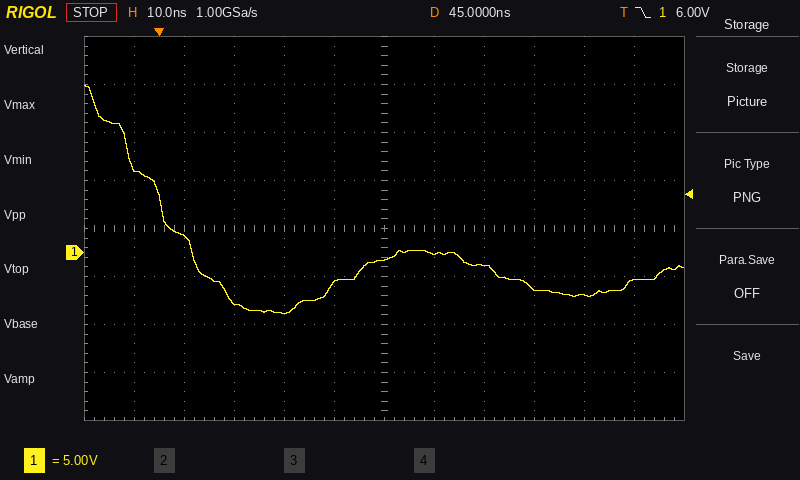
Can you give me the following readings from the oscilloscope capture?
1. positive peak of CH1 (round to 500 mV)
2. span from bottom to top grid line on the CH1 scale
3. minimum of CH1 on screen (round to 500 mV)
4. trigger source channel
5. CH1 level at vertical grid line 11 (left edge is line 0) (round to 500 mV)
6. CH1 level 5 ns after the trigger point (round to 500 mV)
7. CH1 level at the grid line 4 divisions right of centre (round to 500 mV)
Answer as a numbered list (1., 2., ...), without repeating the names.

1. 17.5 V
2. 40 V
3. -6.5 V
4. CH1
5. -3.0 V
6. 1.5 V
7. -4.5 V
